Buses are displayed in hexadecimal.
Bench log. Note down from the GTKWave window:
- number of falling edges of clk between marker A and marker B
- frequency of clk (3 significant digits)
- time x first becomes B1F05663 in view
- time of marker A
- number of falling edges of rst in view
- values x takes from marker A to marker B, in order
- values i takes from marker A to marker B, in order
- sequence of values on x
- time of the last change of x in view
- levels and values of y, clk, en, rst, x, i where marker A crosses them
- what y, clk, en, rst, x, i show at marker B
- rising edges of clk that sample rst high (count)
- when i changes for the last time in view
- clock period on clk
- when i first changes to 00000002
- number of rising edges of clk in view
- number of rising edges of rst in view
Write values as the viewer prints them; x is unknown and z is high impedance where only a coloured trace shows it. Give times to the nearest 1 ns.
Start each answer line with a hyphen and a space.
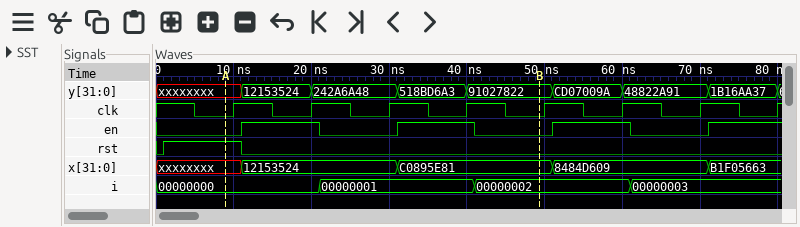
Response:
- 4
- 100 MHz
- 71 ns
- 9 ns
- 1
- xxxxxxxx, 12153524, C0895E81
- 00000000, 00000001, 00000002
- xxxxxxxx, 12153524, C0895E81, 8484D609, B1F05663
- 71 ns
- y=xxxxxxxx, clk=0, en=0, rst=1, x=xxxxxxxx, i=00000000
- y=91027822, clk=0, en=0, rst=0, x=C0895E81, i=00000002
- 1
- 61 ns
- 10 ns
- 41 ns
- 8
- 1
